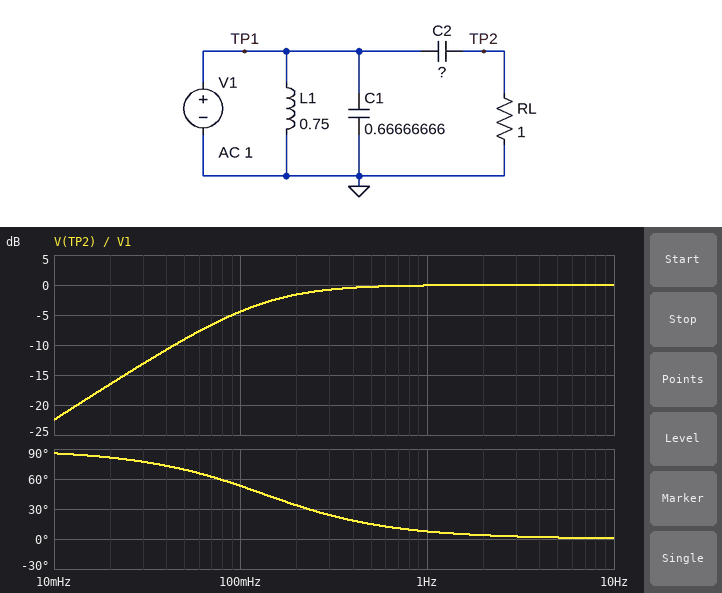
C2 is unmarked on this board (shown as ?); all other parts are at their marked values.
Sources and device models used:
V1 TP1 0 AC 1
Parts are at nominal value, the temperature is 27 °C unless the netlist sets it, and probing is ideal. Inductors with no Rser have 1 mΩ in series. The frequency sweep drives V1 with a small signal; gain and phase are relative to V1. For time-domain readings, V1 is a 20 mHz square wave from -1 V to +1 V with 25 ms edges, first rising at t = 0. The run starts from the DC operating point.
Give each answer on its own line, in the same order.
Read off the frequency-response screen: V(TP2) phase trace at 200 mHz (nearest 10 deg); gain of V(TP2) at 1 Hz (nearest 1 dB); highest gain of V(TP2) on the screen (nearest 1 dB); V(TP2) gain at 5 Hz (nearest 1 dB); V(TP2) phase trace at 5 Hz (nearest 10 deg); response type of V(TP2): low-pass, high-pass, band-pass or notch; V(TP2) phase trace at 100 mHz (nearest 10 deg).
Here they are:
30 deg
0 dB
0 dB
0 dB
0 deg
high-pass
50 deg
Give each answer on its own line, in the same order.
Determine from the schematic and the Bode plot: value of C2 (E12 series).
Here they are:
1.2 F
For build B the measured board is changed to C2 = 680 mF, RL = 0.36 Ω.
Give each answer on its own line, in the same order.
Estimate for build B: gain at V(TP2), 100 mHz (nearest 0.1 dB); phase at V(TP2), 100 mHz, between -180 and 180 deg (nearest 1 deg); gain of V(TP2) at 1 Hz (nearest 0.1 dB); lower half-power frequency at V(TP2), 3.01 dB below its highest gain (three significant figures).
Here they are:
-16.4 dB
81 deg
-1.5 dB
650 mHz
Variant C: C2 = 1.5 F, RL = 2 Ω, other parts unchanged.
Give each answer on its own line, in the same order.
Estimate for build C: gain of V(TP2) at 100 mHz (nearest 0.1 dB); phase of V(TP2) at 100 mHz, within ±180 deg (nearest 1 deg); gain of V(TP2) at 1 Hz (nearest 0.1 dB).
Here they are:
-1.1 dB
28 deg
0 dB
